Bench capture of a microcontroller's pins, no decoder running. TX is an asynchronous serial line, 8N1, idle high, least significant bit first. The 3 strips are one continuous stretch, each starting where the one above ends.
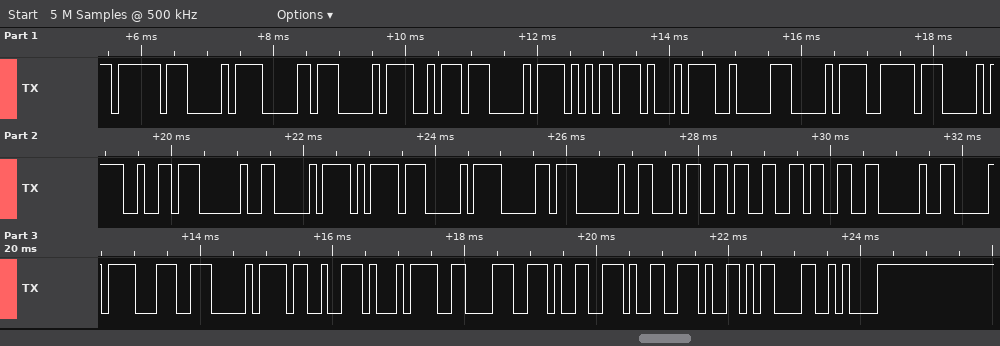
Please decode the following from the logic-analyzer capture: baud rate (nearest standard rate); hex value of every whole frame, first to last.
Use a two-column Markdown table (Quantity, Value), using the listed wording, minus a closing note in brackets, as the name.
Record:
| Quantity | Value |
|---|---|
| baud rate | 9600 baud |
| hex value of every whole frame, first to last | BF D0 B0 D0 BA D0 B5 D1 82 D0 BE D0 B2 20 D0 BD D0 B0 20 34 33 33 20 D0 9C D0 93 D1 86 2E 2E 2E 0D 0A |
